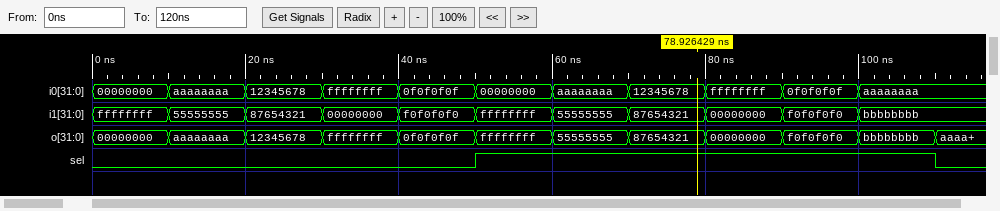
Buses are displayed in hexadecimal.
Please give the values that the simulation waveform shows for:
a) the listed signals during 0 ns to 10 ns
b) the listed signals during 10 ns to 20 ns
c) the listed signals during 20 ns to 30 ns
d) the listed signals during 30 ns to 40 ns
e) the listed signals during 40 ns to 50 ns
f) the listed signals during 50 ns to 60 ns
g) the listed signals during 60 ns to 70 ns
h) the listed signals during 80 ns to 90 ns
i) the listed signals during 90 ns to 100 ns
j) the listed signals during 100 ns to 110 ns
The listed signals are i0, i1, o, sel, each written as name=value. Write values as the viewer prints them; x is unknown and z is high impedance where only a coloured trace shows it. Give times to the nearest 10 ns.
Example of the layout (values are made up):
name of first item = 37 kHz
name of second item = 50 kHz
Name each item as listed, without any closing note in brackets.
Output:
the listed signals during 0 ns to 10 ns = i0=00000000, i1=ffffffff, o=00000000, sel=0
the listed signals during 10 ns to 20 ns = i0=aaaaaaaa, i1=55555555, o=aaaaaaaa, sel=0
the listed signals during 20 ns to 30 ns = i0=12345678, i1=87654321, o=12345678, sel=0
the listed signals during 30 ns to 40 ns = i0=ffffffff, i1=00000000, o=ffffffff, sel=0
the listed signals during 40 ns to 50 ns = i0=0f0f0f0f, i1=f0f0f0f0, o=0f0f0f0f, sel=0
the listed signals during 50 ns to 60 ns = i0=00000000, i1=ffffffff, o=ffffffff, sel=1
the listed signals during 60 ns to 70 ns = i0=aaaaaaaa, i1=55555555, o=55555555, sel=1
the listed signals during 80 ns to 90 ns = i0=ffffffff, i1=00000000, o=00000000, sel=1
the listed signals during 90 ns to 100 ns = i0=0f0f0f0f, i1=f0f0f0f0, o=f0f0f0f0, sel=1
the listed signals during 100 ns to 110 ns = i0=aaaaaaaa, i1=bbbbbbbb, o=bbbbbbbb, sel=1
